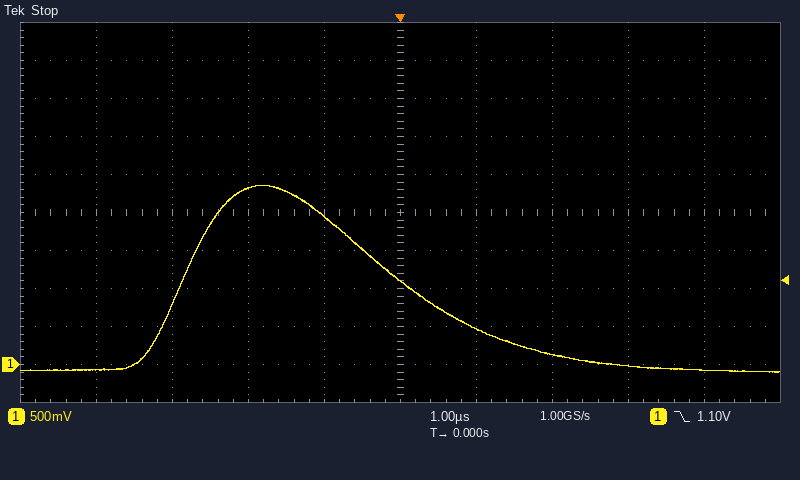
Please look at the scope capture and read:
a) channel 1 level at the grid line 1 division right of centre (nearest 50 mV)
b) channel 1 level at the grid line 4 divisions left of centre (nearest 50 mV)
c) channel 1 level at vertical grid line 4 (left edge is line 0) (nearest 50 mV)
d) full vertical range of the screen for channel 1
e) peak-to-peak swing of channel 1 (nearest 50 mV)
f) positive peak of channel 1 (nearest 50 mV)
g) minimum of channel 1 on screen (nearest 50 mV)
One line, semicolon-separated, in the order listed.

450 mV; -50 mV; 1.95 V; 5 V; 2.45 V; 2.35 V; -100 mV
